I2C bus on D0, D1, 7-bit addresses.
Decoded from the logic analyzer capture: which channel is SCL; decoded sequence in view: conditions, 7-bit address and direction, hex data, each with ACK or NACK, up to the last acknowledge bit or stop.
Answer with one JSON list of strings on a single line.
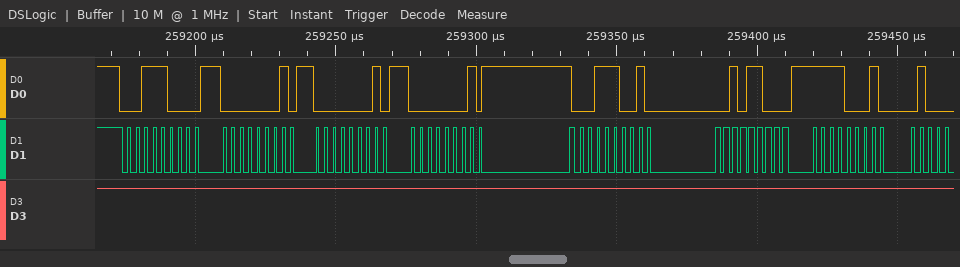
["D1", "start, address 1C write ACK, 01 ACK, 01 ACK, 01 ACK, repeated start, address 1C read ACK, 2C ACK, F1 ACK"]
